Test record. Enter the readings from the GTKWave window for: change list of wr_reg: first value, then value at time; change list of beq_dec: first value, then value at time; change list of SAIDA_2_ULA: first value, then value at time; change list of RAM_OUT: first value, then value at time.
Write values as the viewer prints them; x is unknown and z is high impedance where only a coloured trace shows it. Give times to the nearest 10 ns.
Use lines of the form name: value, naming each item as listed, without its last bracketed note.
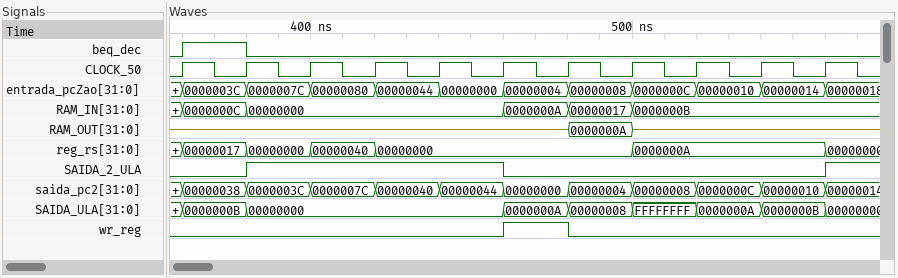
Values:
change list of wr_reg: first value, then value at time: 0, 1 at 460 ns, 0 at 480 ns
change list of beq_dec: first value, then value at time: 0, 1 at 360 ns, 0 at 380 ns
change list of SAIDA_2_ULA: first value, then value at time: 0, 1 at 380 ns, 0 at 460 ns, 1 at 560 ns
change list of RAM_OUT: first value, then value at time: z, 0000000A at 480 ns, z at 500 ns
